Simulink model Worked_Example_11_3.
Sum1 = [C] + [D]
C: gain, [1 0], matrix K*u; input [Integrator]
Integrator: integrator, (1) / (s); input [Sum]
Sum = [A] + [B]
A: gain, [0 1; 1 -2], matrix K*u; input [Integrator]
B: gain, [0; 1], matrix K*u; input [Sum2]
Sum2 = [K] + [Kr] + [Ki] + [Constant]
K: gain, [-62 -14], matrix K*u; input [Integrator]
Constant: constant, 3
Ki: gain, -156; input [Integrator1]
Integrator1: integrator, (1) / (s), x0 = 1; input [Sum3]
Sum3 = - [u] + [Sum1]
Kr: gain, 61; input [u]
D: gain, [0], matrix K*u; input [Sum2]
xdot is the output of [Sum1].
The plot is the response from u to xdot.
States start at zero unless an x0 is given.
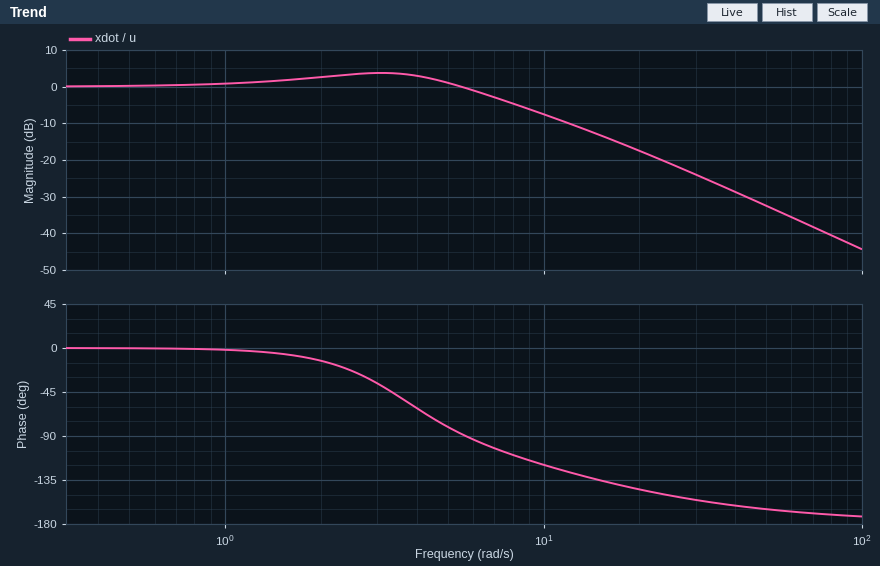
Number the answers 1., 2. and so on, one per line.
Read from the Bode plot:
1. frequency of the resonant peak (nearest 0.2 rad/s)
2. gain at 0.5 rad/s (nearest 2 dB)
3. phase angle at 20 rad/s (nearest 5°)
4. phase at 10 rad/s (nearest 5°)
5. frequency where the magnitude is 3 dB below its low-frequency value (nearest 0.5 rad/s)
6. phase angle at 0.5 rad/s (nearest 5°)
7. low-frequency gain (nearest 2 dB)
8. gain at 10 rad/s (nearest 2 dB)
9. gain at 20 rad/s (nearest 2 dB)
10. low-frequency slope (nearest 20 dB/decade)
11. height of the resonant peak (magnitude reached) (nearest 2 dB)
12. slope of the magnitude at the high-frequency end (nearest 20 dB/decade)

1. 3.0 rad/s
2. 0 dB
3. -145°
4. -120°
5. 7.0 rad/s
6. 0°
7. 0 dB
8. -8 dB
9. -18 dB
10. 0 dB/decade
11. 4 dB
12. -40 dB/decade
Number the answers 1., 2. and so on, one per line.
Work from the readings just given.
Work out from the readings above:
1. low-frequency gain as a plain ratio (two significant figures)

1. 1.0
